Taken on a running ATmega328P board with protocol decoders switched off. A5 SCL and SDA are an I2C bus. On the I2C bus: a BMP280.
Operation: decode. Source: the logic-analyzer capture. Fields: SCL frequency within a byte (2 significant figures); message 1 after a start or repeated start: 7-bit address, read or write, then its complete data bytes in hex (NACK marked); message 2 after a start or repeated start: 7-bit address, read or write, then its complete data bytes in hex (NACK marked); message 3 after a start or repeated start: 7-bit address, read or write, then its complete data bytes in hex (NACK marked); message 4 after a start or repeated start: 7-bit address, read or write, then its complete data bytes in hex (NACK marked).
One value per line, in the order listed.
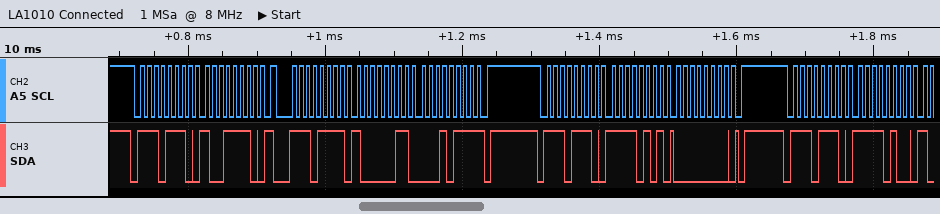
100 kHz
0x77 write: 9E
0x77 read: 83 17 NACK
0x77 write: F5 00
0x77 write: F4
